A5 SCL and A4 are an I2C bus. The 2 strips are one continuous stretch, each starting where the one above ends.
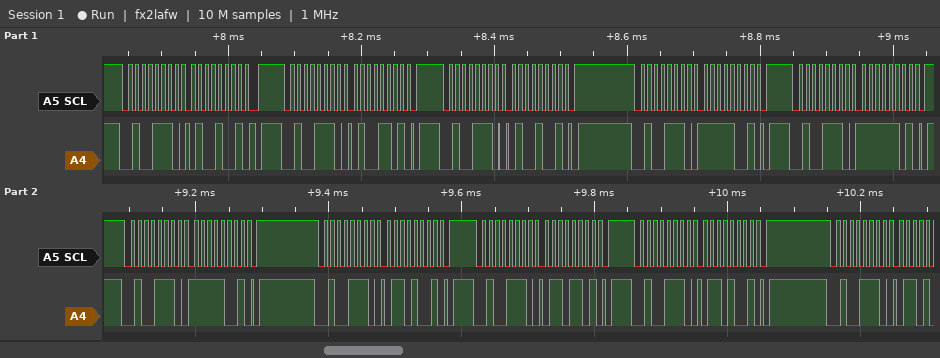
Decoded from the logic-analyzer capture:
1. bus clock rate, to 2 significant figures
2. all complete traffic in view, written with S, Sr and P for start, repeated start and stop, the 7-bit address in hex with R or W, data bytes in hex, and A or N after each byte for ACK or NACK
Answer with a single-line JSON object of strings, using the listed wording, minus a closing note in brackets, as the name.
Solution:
{"bus clock rate, to 2 significant figures": "100 kHz", "all complete traffic in view, written with S, Sr and P for start, repeated start and stop, the 7-bit address in hex with R or W, data bytes in hex, and A or N after each byte for ACK or NACK": "S 27W A 49 A P S 27W A 4D A P S 27W A 49 A P S 27W A F9 A P S 27W A FD A P S 27W A F9 A P S 27W A 69 A P S 27W A 6D A P S 27W A 69 A P S 27W A"}
